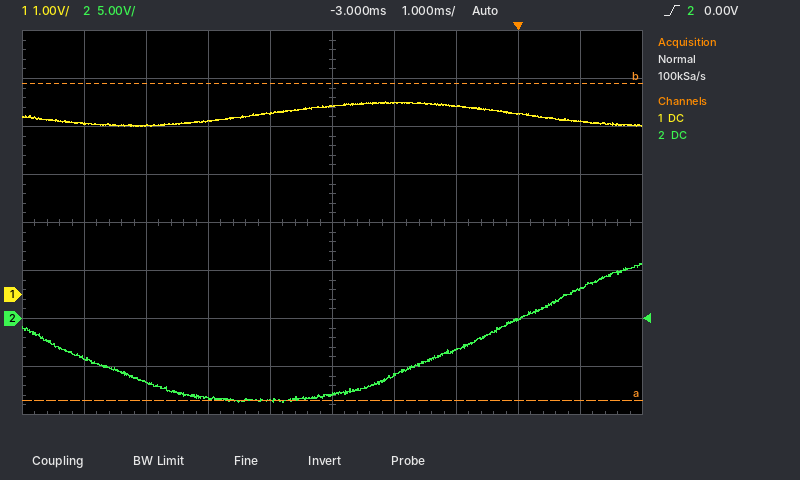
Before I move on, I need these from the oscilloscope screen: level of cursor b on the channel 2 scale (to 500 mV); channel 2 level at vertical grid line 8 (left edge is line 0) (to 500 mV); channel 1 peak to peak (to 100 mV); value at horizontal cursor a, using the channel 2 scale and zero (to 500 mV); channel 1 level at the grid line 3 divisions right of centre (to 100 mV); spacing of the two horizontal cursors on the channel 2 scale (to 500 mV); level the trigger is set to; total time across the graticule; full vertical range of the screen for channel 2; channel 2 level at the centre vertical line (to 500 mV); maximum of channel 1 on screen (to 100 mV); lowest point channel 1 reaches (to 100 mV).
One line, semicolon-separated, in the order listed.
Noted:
24.5 V; 0.0 V; 500 mV; -8.5 V; 3.8 V; 33.0 V; 0.00 V; 10 ms; 40 V; -8.0 V; 4.0 V; 3.5 V
